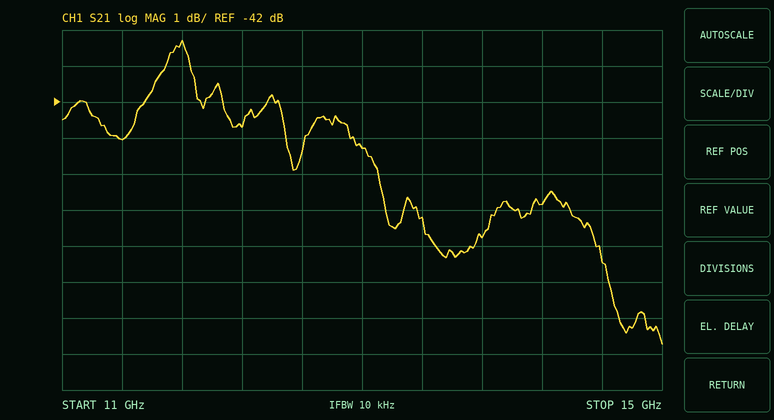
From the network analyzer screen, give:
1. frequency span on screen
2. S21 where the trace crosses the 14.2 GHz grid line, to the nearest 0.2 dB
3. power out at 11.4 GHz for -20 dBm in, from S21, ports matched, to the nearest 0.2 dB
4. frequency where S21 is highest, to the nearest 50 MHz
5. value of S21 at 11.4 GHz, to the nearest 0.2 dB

4 GHz
-44.8 dB
-63.0 dBm
11.80 GHz
-43.0 dB
